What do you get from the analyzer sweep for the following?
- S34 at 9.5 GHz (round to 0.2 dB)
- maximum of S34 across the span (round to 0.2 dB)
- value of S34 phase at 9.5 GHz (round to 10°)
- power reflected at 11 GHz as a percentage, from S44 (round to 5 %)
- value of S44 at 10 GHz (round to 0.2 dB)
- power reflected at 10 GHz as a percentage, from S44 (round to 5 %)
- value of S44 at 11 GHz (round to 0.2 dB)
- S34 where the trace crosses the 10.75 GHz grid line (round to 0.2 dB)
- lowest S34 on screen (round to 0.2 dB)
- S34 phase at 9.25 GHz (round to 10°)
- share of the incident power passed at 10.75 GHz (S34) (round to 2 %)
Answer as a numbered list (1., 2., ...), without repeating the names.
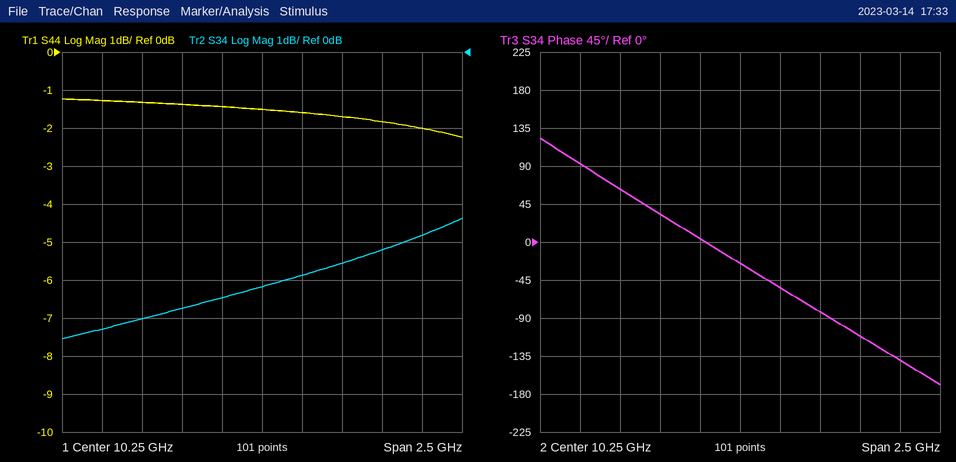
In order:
1. -7.0 dB
2. -4.4 dB
3. 60°
4. 65 %
5. -1.4 dB
6. 70 %
7. -1.8 dB
8. -5.6 dB
9. -7.6 dB
10. 90°
11. 28 %
